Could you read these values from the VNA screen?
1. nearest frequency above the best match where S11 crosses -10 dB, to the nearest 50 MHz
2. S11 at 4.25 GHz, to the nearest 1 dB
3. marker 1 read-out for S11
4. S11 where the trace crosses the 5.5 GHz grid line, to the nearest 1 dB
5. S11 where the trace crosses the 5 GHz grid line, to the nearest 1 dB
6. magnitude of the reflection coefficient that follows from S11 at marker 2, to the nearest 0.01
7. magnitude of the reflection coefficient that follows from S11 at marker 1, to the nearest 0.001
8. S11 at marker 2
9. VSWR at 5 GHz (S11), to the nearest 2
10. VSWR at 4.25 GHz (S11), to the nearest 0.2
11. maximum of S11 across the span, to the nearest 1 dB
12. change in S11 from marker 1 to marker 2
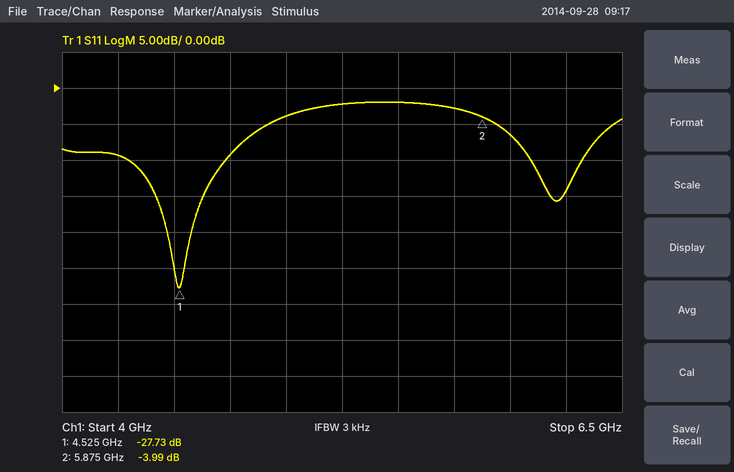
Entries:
4.75 GHz
-9 dB
-27.73 dB
-2 dB
-4 dB
0.63
0.041
-3.99 dB
4
2.0
-2 dB
23.74 dB
